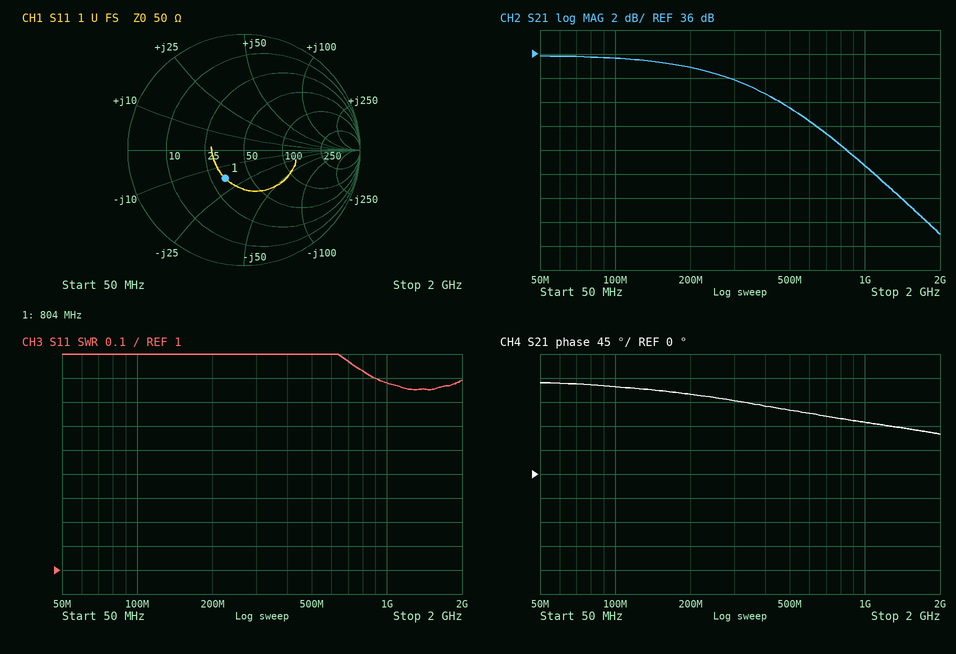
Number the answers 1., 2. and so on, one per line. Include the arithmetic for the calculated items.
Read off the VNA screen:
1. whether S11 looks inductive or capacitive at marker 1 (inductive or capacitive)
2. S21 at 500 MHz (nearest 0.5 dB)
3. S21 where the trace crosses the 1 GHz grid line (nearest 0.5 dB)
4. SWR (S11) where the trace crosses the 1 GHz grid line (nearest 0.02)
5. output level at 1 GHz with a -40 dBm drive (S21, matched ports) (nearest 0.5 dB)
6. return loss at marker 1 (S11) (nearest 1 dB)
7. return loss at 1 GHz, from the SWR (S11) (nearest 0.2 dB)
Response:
1. capacitive
2. 31.5 dB
3. 26.5 dB
4. 1.78
5. -40 dBm + (26.5 dB) = -13.5 dBm
6. 11 dB
7. −20 log10((1.78 − 1)/(1.78 + 1)) ≈ 11.0 dB
